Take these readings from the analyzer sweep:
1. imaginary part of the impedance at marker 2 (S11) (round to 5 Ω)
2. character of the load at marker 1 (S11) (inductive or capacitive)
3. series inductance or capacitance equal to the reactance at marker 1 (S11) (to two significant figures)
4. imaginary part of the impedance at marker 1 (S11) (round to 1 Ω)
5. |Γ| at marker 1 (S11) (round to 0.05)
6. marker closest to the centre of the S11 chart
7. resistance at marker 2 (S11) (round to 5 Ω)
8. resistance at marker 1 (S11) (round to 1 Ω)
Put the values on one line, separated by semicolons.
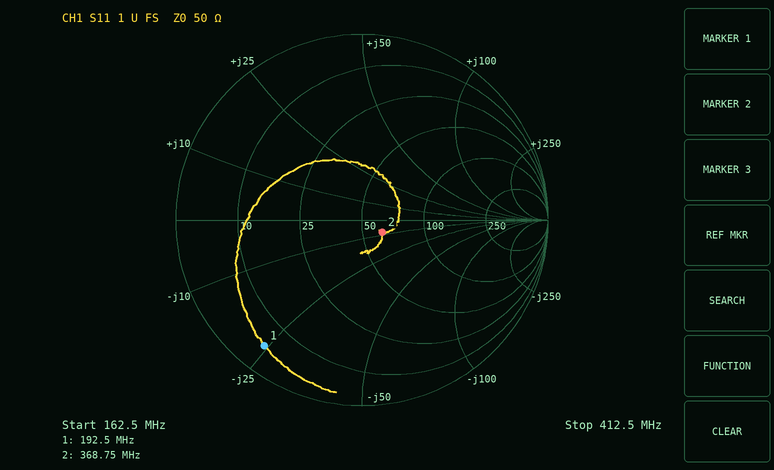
-10 Ω; capacitive; 34 pF; -24 Ω; 0.85; marker 2; 60 Ω; 5 Ω
